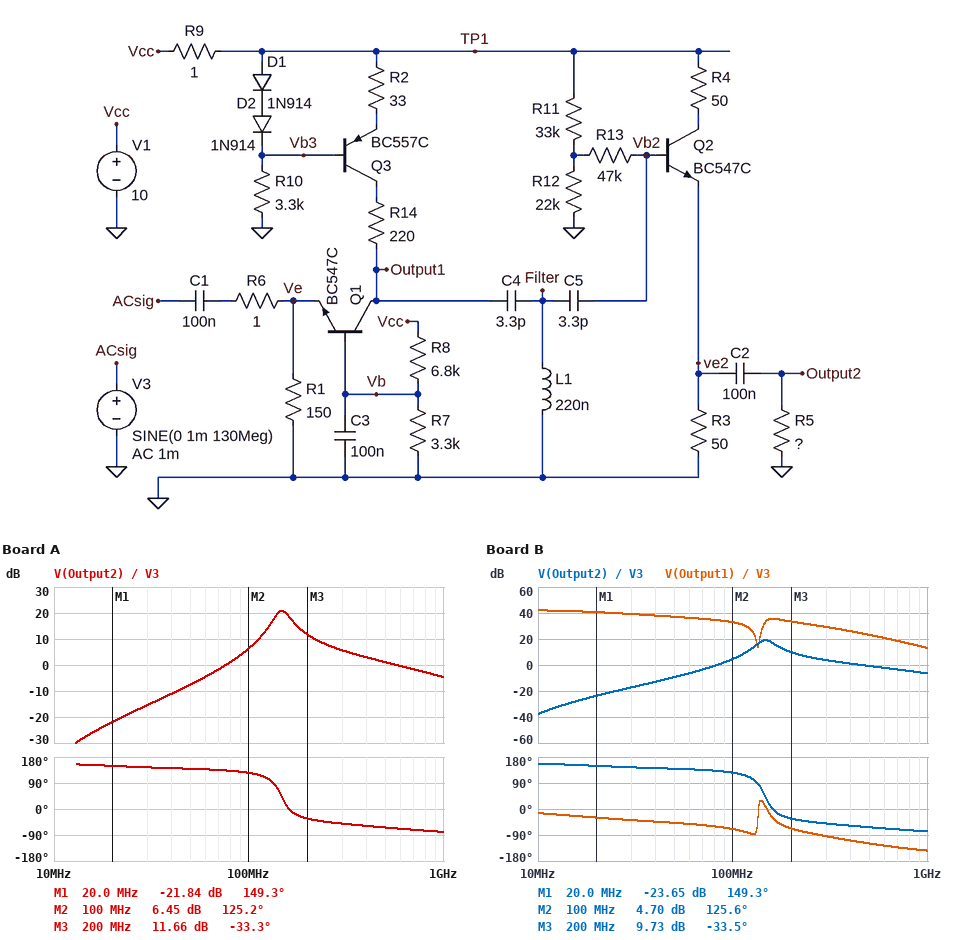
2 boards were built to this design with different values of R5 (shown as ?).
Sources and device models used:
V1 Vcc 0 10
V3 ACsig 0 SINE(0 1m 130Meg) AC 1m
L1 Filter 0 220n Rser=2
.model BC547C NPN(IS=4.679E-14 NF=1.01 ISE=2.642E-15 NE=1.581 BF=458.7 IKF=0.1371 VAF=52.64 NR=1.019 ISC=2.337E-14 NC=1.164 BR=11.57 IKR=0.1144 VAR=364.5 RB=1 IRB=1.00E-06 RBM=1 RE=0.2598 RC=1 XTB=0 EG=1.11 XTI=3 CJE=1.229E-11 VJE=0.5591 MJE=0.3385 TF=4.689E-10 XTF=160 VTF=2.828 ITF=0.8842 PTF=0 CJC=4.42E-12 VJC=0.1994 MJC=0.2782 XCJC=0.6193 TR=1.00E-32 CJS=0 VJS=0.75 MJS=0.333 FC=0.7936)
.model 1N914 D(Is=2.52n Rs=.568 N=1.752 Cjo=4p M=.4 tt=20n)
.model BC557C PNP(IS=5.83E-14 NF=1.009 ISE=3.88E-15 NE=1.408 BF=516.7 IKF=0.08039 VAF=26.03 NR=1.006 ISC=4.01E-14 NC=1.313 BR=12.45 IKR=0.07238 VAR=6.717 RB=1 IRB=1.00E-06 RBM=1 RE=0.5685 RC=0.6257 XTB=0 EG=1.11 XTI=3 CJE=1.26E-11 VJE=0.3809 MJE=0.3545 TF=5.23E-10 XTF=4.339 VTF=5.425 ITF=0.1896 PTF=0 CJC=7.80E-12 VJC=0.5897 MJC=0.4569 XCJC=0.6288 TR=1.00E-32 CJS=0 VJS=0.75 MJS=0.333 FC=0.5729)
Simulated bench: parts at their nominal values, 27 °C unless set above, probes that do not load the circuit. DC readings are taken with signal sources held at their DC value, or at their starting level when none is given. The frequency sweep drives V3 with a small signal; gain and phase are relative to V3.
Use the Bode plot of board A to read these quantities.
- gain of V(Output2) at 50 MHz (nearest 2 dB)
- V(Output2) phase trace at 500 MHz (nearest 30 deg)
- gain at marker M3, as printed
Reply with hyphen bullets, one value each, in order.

- -8 dB
- -60 deg
- 11.66 dB
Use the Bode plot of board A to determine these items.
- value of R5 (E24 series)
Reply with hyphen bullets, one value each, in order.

- 22 Ω
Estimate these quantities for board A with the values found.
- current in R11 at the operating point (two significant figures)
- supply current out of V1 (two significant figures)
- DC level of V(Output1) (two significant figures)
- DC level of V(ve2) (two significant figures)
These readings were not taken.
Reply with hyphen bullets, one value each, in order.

- 200 µA
- 39 mA
- 5.7 V
- 920 mV
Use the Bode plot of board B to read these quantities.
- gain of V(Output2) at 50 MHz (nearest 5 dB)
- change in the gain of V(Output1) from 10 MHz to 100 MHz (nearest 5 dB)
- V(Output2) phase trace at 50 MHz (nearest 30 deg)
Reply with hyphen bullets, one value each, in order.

- -10 dB
- -10 dB
- 150 deg
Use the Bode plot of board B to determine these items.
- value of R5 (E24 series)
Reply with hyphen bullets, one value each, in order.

- 16 Ω
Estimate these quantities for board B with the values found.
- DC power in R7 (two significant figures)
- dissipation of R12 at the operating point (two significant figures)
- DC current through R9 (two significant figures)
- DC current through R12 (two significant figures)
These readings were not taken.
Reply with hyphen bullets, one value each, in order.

- 3.1 mW
- 550 µW
- 38 mA
- 160 µA
